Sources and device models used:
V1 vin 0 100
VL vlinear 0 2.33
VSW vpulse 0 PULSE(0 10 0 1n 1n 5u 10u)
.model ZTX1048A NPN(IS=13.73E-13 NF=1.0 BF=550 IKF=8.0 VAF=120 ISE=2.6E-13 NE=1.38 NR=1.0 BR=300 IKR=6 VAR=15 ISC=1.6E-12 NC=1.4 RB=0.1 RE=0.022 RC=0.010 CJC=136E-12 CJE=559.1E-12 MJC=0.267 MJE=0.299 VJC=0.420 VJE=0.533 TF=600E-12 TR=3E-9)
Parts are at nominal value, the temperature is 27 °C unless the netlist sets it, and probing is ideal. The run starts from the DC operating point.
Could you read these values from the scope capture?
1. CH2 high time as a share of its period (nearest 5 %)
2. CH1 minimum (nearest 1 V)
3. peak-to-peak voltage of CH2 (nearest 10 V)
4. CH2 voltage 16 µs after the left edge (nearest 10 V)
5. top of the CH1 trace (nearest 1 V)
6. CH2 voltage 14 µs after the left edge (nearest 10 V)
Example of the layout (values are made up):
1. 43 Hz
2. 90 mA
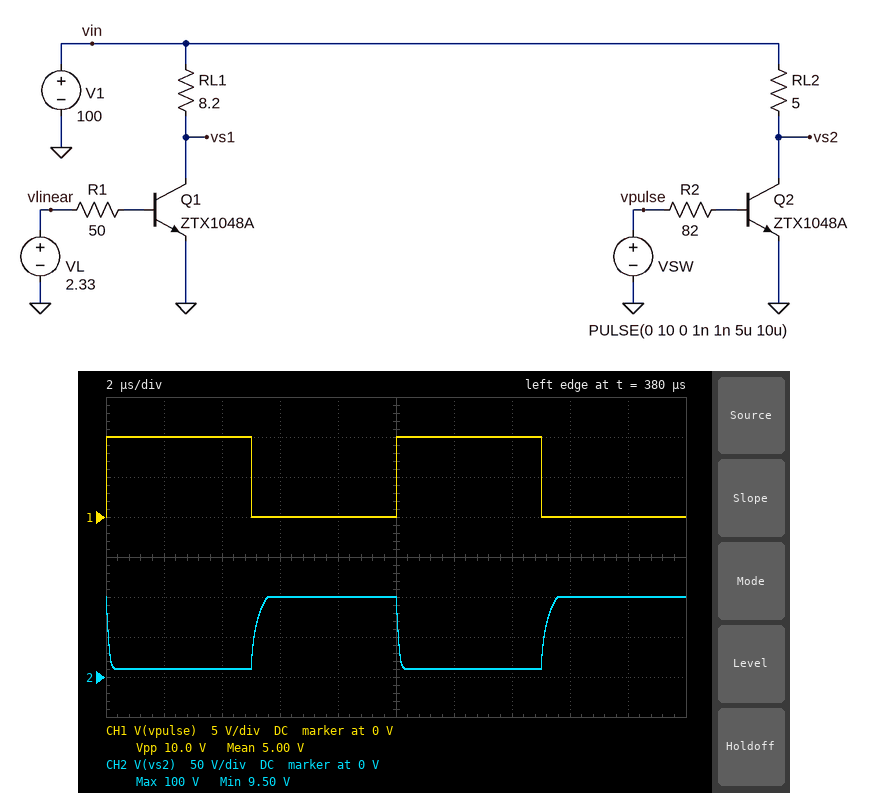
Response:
1. 50 %
2. 0 V
3. 90 V
4. 100 V
5. 10 V
6. 10 V
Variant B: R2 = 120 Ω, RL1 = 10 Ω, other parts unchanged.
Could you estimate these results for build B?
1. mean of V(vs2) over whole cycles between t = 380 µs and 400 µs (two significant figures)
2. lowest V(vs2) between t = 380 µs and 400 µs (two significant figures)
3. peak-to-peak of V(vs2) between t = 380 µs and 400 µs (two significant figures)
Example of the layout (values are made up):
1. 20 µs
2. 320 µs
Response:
1. 60 V
2. 21 V
3. 79 V
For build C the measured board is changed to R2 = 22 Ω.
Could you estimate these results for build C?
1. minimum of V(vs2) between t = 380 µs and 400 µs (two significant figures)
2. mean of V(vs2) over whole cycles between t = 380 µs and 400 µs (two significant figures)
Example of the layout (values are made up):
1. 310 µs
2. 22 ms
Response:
1. 670 mV
2. 46 V
